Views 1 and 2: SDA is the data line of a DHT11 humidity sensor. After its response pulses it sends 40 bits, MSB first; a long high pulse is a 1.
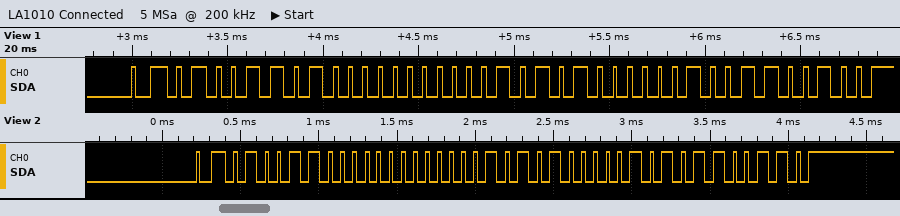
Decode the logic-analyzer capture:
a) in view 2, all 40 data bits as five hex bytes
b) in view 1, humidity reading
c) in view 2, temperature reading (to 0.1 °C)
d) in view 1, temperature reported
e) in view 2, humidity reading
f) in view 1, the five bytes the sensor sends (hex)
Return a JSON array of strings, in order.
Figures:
["4C 00 15 05 66", "77 %", "21.5 °C", "21.2 °C", "76 %", "4D 00 15 02 64"]
